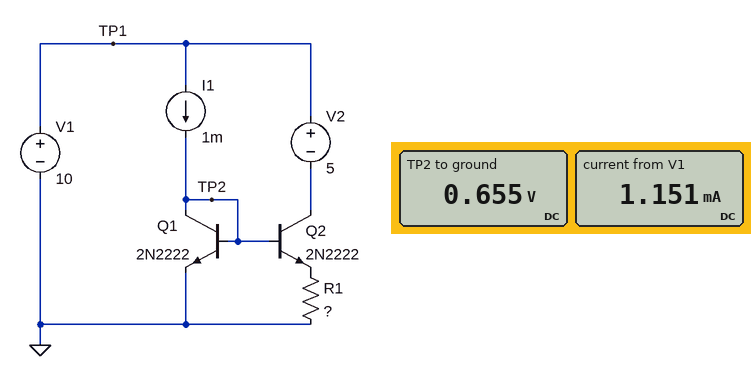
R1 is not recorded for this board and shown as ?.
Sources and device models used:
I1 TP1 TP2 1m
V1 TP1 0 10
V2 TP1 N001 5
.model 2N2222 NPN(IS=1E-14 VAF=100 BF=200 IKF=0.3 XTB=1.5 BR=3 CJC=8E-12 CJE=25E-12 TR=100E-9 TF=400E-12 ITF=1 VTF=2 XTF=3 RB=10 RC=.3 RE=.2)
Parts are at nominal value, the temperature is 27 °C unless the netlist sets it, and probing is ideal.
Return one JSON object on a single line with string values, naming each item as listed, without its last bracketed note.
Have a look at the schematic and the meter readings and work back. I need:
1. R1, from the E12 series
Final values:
{"R1, from the E12 series": "330 Ω"}
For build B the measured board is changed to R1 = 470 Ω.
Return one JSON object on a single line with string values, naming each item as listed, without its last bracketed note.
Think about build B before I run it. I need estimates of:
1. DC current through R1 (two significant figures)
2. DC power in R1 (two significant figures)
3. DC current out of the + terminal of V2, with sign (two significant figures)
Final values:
{"DC current through R1": "120 µA", "DC power in R1": "6.7 µW", "DC current out of the + terminal of V2, with sign": "-120 µA"}
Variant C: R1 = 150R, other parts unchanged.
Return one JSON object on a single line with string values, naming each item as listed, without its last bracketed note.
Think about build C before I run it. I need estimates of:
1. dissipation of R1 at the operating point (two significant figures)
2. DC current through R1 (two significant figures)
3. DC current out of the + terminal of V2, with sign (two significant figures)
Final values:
{"dissipation of R1 at the operating point": "9.3 µW", "DC current through R1": "250 µA", "DC current out of the + terminal of V2, with sign": "-250 µA"}
